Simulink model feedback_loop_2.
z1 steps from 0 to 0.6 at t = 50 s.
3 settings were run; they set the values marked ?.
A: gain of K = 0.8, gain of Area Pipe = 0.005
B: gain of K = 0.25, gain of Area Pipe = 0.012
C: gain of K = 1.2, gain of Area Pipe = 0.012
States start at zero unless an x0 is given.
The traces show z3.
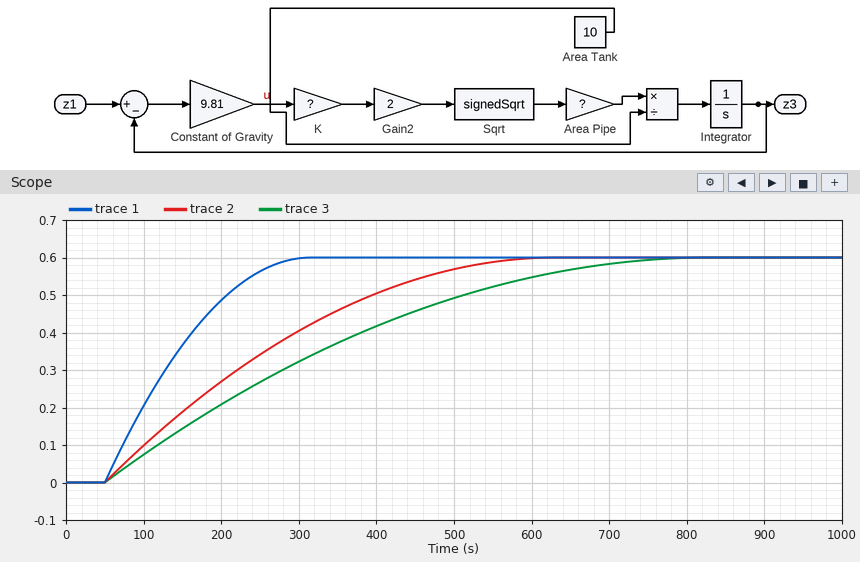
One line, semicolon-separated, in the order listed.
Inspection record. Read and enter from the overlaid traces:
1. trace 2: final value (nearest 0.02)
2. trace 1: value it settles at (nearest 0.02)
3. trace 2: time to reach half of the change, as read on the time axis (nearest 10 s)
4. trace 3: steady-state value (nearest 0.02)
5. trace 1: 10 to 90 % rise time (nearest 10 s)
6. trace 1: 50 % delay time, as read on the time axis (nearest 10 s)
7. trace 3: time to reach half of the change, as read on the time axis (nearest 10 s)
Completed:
0.60; 0.60; 220 s; 0.60; 170 s; 130 s; 280 s
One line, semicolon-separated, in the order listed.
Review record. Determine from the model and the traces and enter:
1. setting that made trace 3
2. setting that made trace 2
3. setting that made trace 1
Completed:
A; B; C
